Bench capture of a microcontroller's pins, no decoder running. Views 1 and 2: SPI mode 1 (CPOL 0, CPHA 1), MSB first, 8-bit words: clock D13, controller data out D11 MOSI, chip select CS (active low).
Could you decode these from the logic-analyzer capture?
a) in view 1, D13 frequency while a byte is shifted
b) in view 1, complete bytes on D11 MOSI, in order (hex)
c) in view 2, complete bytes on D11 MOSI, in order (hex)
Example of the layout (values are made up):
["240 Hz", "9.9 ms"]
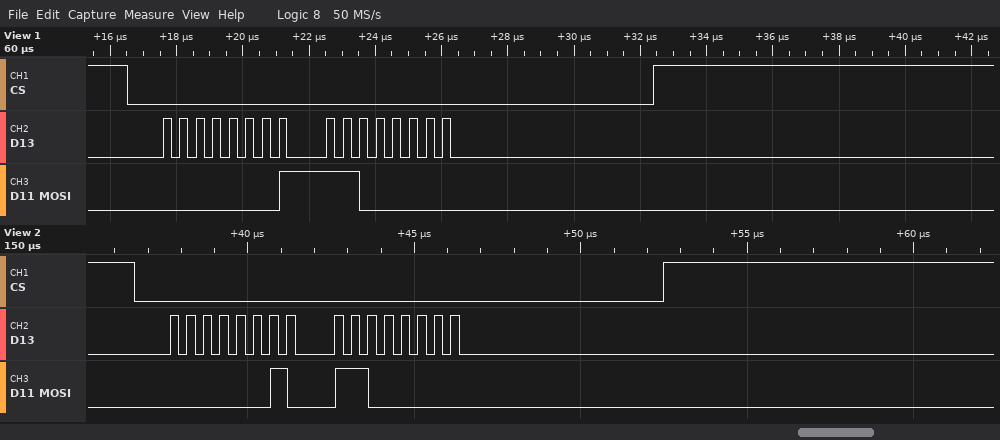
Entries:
["2 MHz", "01 C0", "02 C0"]
